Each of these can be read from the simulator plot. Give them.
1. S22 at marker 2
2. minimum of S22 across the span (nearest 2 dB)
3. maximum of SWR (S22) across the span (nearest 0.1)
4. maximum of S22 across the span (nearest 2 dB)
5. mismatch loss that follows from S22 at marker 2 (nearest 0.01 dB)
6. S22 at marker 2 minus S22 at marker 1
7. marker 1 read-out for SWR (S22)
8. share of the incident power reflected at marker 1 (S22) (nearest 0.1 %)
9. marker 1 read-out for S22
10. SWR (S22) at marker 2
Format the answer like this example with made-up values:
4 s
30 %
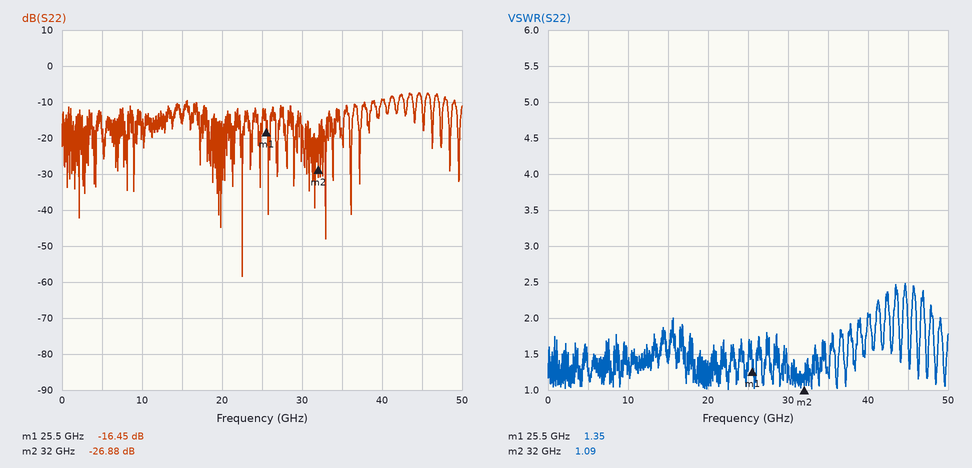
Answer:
-26.88 dB
-58 dB
2.5
-8 dB
0.01 dB
-10.43 dB
1.35
2.3 %
-16.45 dB
1.09
